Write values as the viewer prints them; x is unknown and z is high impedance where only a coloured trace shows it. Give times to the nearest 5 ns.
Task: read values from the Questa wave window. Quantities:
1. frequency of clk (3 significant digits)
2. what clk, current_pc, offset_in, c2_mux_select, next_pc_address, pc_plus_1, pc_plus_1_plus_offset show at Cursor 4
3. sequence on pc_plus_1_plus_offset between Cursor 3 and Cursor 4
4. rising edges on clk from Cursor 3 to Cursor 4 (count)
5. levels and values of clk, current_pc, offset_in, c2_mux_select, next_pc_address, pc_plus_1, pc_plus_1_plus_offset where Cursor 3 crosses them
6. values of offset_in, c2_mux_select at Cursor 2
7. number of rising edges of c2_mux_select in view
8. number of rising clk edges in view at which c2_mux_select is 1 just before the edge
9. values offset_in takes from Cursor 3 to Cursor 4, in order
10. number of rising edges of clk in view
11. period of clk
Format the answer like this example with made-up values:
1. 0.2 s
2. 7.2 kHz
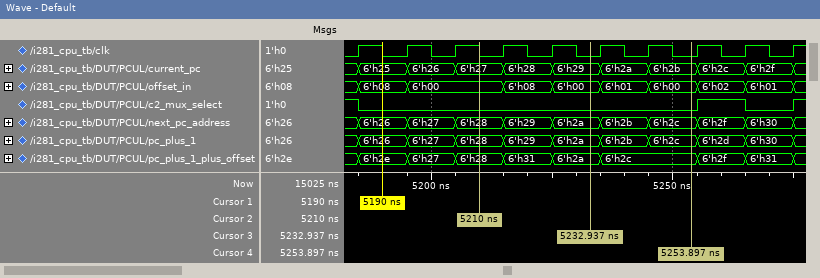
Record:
1. 100 MHz
2. clk=0, current_pc=6'h2b, offset_in=6'h00, c2_mux_select=0, next_pc_address=6'h2c, pc_plus_1=6'h2c, pc_plus_1_plus_offset=6'h2c
3. 6'h2a, 6'h2c
4. 2
5. clk=0, current_pc=6'h29, offset_in=6'h00, c2_mux_select=0, next_pc_address=6'h2a, pc_plus_1=6'h2a, pc_plus_1_plus_offset=6'h2a
6. offset_in=6'h00, c2_mux_select=0
7. 2
8. 2
9. 6'h00, 6'h01, 6'h00
10. 10
11. 10 ns
